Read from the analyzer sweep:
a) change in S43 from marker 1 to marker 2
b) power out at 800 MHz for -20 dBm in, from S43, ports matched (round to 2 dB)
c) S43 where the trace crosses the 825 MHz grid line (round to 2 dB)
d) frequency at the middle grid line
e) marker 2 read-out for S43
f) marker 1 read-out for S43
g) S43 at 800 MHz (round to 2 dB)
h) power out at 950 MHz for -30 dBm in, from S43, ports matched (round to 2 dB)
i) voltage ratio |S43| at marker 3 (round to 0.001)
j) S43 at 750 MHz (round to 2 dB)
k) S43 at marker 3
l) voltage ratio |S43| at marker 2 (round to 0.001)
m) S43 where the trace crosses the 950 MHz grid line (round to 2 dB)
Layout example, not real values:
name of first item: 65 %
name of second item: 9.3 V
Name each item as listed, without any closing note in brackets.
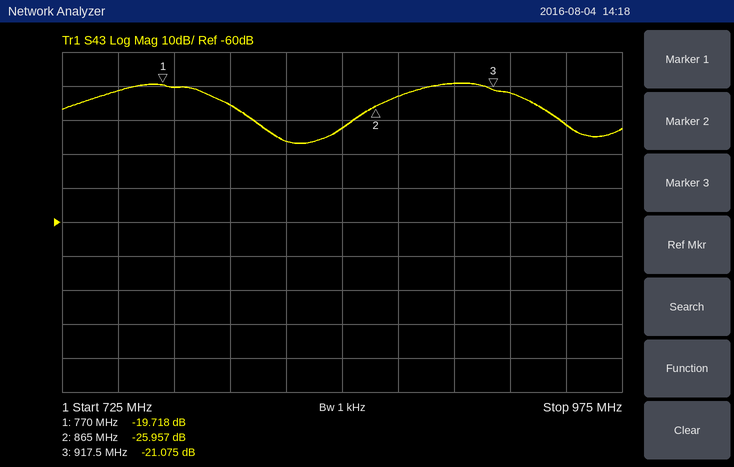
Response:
change in S43 from marker 1 to marker 2: -6.239 dB
power out at 800 MHz for -20 dBm in, from S43, ports matched: -46 dBm
S43 where the trace crosses the 825 MHz grid line: -36 dB
frequency at the middle grid line: 850 MHz
marker 2 read-out for S43: -25.957 dB
marker 1 read-out for S43: -19.718 dB
S43 at 800 MHz: -26 dB
power out at 950 MHz for -30 dBm in, from S43, ports matched: -62 dBm
voltage ratio |S43| at marker 3: 0.088
S43 at 750 MHz: -22 dB
S43 at marker 3: -21.075 dB
voltage ratio |S43| at marker 2: 0.050
S43 where the trace crosses the 950 MHz grid line: -32 dB
